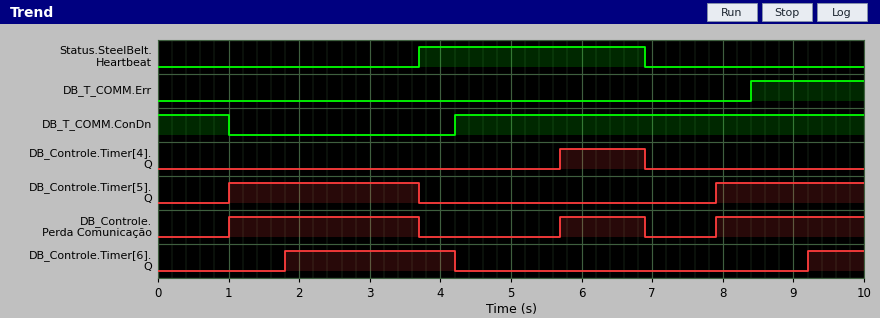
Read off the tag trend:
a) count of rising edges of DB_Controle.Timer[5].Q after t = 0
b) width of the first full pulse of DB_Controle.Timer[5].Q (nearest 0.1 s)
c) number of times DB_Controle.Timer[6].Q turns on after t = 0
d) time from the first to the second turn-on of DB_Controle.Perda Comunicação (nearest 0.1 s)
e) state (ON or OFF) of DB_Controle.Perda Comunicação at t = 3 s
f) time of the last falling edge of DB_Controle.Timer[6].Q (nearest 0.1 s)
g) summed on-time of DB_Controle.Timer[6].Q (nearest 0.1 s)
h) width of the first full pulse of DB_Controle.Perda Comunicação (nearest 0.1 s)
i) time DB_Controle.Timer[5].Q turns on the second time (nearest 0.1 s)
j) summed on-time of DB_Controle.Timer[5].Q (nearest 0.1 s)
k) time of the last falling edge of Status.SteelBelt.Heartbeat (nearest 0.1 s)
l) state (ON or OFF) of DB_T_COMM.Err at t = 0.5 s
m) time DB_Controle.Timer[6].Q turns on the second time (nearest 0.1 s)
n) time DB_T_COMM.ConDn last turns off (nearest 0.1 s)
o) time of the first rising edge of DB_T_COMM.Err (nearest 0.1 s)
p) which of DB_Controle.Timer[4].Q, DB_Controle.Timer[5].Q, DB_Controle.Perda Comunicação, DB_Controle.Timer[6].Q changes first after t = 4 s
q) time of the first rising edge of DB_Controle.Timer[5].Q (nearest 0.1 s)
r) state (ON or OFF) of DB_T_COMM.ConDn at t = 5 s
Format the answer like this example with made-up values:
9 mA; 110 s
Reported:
2; 2.7 s; 2; 4.7 s; ON; 4.2 s; 3.2 s; 2.7 s; 7.9 s; 4.8 s; 6.9 s; OFF; 9.2 s; 1.0 s; 8.4 s; DB_Controle.Timer[6].Q; 1.0 s; ON
